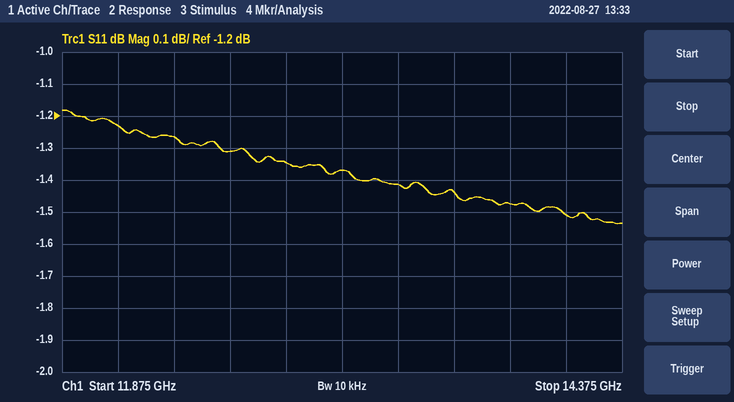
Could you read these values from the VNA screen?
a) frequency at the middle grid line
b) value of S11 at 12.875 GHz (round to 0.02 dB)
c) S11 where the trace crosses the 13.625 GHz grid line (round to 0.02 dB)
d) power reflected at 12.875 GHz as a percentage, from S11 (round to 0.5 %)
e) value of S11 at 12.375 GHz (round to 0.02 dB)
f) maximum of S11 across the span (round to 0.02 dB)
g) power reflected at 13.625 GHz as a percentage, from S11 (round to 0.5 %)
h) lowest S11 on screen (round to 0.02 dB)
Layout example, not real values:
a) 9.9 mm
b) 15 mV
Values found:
a) 13.125 GHz
b) -1.34 dB
c) -1.44 dB
d) 73.5 %
e) -1.26 dB
f) -1.18 dB
g) 72.0 %
h) -1.54 dB
